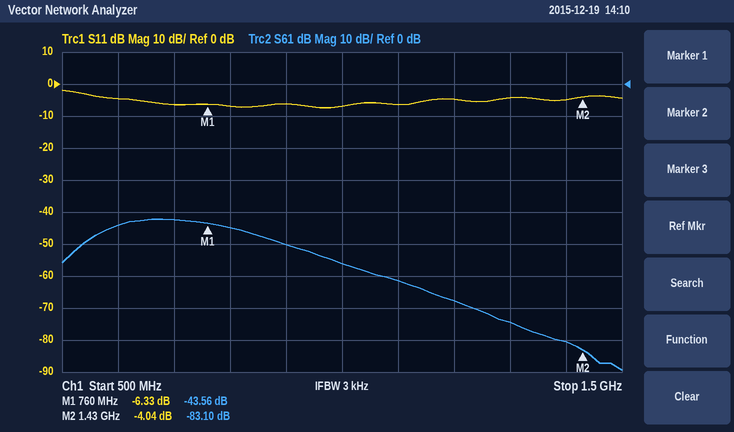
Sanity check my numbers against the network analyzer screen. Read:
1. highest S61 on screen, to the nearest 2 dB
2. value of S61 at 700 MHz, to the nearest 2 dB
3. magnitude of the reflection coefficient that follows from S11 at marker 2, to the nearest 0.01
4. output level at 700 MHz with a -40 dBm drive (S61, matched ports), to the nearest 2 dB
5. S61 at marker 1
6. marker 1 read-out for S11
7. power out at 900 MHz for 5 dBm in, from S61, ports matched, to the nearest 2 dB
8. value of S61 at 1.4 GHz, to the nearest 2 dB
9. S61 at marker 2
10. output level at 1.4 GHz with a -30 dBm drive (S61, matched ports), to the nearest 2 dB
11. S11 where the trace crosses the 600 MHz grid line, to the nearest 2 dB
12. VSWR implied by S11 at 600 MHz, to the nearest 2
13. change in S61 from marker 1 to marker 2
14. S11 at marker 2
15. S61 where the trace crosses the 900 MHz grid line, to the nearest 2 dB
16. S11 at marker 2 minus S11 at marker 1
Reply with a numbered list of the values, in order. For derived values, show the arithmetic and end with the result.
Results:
1. -42 dB
2. -42 dB
3. 10^(-4.04/20) ≈ 0.63
4. -40 dBm + (-42 dB) = -82 dBm
5. -43.56 dB
6. -6.33 dB
7. 5 dBm + (-50 dB) = -46 dBm
8. -80 dB
9. -83.10 dB
10. -30 dBm + (-80 dB) = -110 dBm
11. -4 dB
12. |Γ| = 10^(-4/20) = 0.6310; VSWR = (1 + 0.6310)/(1 − 0.6310) ≈ 4
13. -83.1 − (-43.56) = -39.54 dB
14. -4.04 dB
15. -50 dB
16. -4.04 − (-6.33) = 2.29 dB
